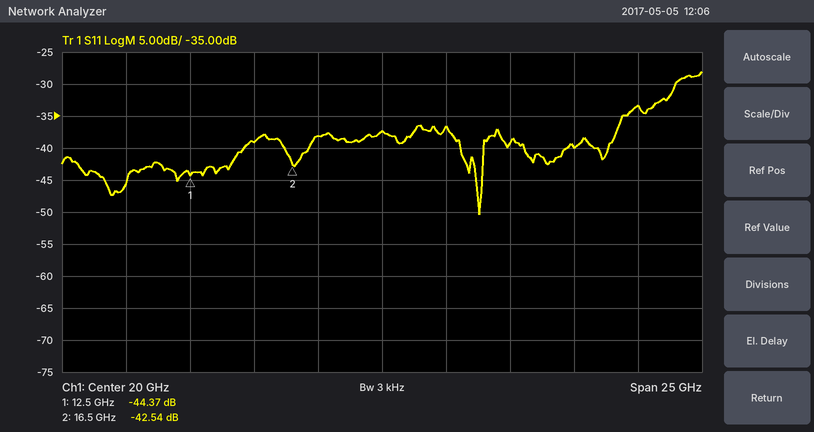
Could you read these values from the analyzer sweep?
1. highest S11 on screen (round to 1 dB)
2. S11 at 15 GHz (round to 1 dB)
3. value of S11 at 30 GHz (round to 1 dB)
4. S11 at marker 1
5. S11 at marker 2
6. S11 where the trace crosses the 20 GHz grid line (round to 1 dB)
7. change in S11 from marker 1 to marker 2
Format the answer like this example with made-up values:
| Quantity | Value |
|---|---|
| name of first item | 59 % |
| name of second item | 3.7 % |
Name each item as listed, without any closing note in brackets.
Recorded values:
| Quantity | Value |
|---|---|
| highest S11 on screen | -28 dB |
| S11 at 15 GHz | -39 dB |
| value of S11 at 30 GHz | -33 dB |
| S11 at marker 1 | -44.37 dB |
| S11 at marker 2 | -42.54 dB |
| S11 where the trace crosses the 20 GHz grid line | -37 dB |
| change in S11 from marker 1 to marker 2 | 1.83 dB |
